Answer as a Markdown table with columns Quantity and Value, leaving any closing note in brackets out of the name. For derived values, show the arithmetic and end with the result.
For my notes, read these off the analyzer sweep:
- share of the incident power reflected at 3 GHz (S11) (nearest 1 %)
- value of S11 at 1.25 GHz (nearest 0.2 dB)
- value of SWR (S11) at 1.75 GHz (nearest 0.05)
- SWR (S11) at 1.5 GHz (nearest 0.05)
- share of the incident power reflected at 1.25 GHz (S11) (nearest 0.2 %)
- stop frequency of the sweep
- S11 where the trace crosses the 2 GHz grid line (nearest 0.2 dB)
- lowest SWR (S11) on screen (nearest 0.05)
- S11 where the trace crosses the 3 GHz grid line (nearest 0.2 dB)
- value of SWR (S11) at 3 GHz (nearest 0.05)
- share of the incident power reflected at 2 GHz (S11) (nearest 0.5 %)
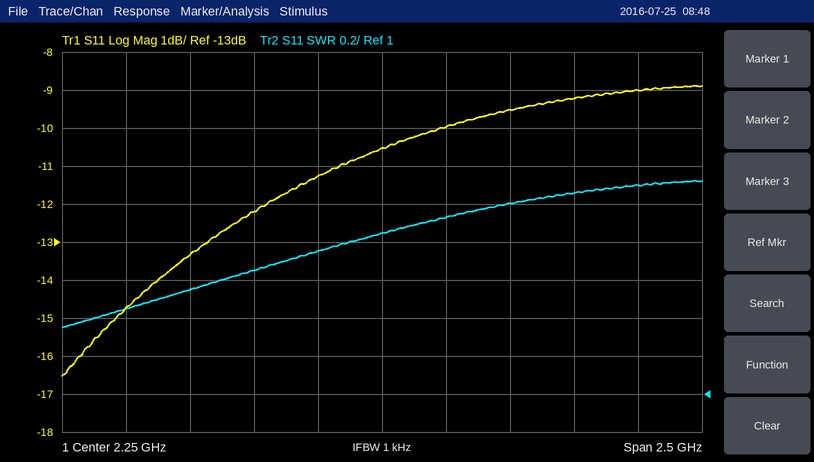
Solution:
| Quantity | Value |
|---|---|
| share of the incident power reflected at 3 GHz (S11) | 10^(-9.2/10) ≈ 12 % |
| value of S11 at 1.25 GHz | -14.8 dB |
| value of SWR (S11) at 1.75 GHz | 1.65 |
| SWR (S11) at 1.5 GHz | 1.55 |
| share of the incident power reflected at 1.25 GHz (S11) | 10^(-14.8/10) ≈ 3.31 %, so 3.4 % to the nearest 0.2 % |
| stop frequency of the sweep | 3.5 GHz |
| S11 where the trace crosses the 2 GHz grid line | -11.2 dB |
| lowest SWR (S11) on screen | 1.35 |
| S11 where the trace crosses the 3 GHz grid line | -9.2 dB |
| value of SWR (S11) at 3 GHz | 2.05 |
| share of the incident power reflected at 2 GHz (S11) | 10^(-11.2/10) ≈ 7.59 %, so 7.5 % to the nearest 0.5 % |
